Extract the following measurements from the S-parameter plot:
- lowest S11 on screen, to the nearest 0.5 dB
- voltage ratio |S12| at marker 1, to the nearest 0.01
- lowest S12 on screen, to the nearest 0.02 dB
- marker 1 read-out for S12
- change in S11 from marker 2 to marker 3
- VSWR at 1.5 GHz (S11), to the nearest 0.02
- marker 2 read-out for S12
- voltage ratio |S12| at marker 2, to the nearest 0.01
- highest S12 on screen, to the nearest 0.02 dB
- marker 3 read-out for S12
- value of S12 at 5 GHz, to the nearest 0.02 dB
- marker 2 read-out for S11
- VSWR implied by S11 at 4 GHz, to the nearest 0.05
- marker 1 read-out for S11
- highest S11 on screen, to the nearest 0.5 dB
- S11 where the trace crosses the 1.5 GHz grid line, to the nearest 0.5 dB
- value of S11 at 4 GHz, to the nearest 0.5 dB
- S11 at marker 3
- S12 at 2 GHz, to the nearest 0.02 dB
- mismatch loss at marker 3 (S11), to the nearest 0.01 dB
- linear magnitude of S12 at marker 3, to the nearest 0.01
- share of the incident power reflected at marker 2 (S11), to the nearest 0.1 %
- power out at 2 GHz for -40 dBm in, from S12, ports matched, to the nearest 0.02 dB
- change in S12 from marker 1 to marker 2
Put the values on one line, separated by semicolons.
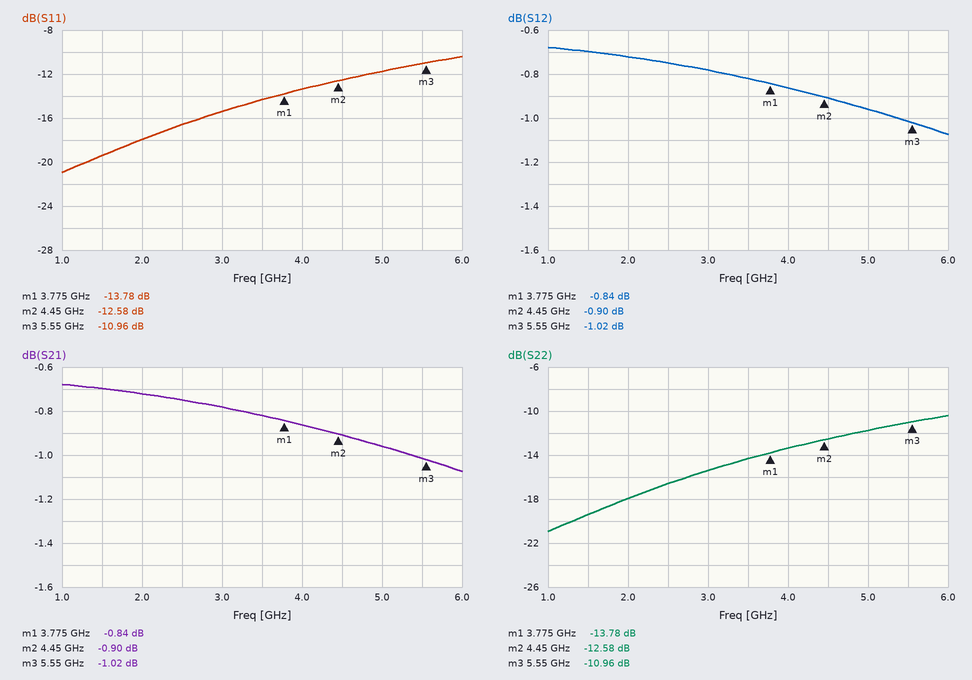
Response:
-21.0 dB; 0.91; -1.08 dB; -0.84 dB; 1.62 dB; 1.24; -0.90 dB; 0.90; -0.68 dB; -1.02 dB; -0.96 dB; -12.58 dB; 1.55; -13.78 dB; -10.5 dB; -19.5 dB; -13.5 dB; -10.96 dB; -0.72 dB; 0.36 dB; 0.89; 5.5 %; -40.72 dBm; -0.06 dB
